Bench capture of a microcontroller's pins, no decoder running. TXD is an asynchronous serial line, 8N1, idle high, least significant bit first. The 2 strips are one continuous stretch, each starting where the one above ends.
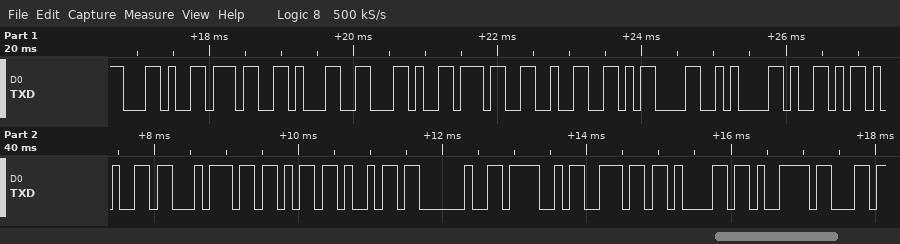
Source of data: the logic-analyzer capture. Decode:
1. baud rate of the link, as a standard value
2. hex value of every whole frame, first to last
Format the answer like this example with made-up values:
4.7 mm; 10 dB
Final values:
9600 baud; 2C 37 31 2C 37 32 0D 0A 59 65 74 6B 69 20 4F 6E 61 79
